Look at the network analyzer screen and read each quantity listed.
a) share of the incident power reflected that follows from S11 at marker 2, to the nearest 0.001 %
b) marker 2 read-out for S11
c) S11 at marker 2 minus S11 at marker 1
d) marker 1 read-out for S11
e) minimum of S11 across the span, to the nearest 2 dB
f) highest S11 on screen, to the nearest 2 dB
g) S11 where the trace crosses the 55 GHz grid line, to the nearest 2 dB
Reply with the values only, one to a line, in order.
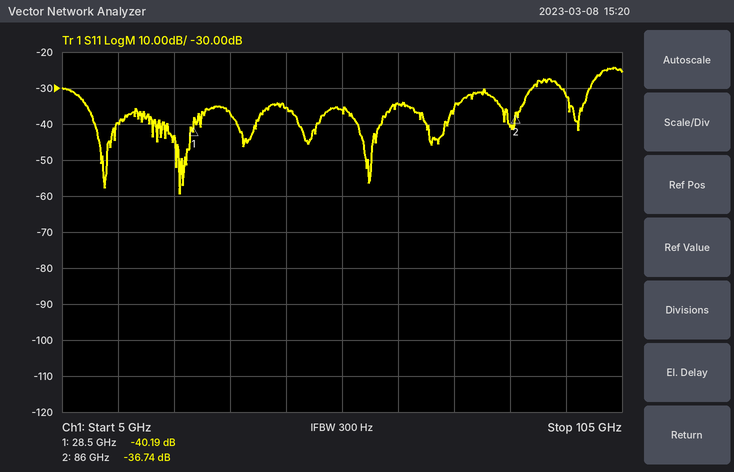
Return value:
0.021 %
-36.74 dB
3.45 dB
-40.19 dB
-60 dB
-24 dB
-36 dB
